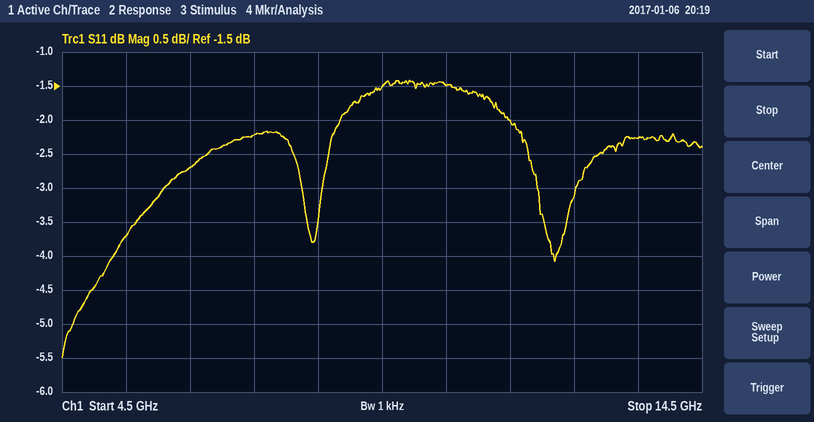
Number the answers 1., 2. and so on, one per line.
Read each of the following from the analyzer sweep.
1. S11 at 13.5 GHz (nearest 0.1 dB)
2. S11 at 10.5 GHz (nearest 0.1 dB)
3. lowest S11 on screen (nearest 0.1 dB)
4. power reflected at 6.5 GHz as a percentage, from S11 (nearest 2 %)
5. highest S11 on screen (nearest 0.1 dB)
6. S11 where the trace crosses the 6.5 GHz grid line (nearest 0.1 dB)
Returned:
1. -2.3 dB
2. -1.5 dB
3. -5.5 dB
4. 54 %
5. -1.4 dB
6. -2.7 dB
